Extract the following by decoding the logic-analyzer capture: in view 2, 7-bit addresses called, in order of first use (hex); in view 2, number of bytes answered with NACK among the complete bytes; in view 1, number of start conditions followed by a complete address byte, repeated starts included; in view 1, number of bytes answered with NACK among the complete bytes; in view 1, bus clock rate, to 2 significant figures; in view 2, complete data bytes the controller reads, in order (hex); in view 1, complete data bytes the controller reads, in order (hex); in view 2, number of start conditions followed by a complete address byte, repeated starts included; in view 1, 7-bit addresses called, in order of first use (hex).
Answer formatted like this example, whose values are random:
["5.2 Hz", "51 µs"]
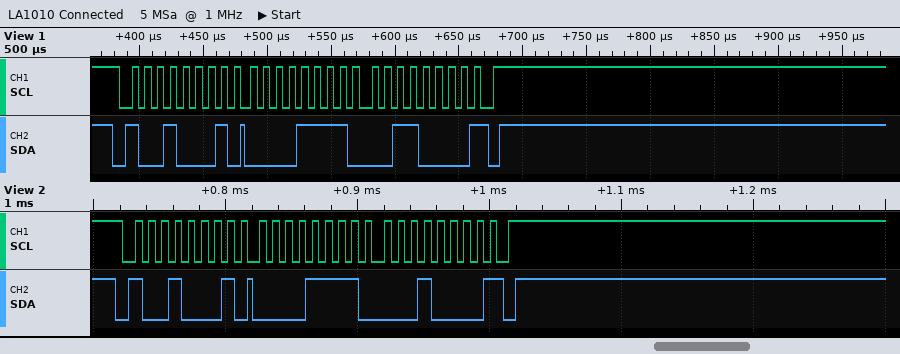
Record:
["0x48", "1", "1", "1", "100 kHz", "0F 10", "0F 30", "1", "0x48"]
